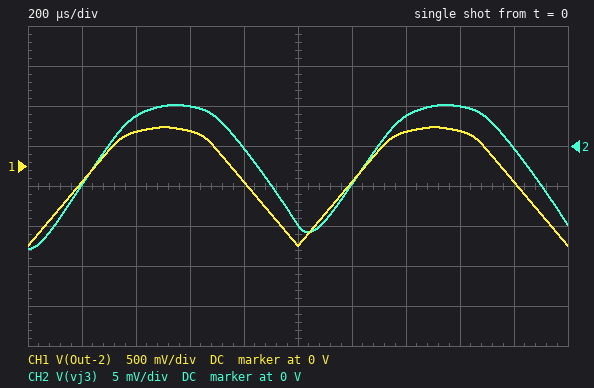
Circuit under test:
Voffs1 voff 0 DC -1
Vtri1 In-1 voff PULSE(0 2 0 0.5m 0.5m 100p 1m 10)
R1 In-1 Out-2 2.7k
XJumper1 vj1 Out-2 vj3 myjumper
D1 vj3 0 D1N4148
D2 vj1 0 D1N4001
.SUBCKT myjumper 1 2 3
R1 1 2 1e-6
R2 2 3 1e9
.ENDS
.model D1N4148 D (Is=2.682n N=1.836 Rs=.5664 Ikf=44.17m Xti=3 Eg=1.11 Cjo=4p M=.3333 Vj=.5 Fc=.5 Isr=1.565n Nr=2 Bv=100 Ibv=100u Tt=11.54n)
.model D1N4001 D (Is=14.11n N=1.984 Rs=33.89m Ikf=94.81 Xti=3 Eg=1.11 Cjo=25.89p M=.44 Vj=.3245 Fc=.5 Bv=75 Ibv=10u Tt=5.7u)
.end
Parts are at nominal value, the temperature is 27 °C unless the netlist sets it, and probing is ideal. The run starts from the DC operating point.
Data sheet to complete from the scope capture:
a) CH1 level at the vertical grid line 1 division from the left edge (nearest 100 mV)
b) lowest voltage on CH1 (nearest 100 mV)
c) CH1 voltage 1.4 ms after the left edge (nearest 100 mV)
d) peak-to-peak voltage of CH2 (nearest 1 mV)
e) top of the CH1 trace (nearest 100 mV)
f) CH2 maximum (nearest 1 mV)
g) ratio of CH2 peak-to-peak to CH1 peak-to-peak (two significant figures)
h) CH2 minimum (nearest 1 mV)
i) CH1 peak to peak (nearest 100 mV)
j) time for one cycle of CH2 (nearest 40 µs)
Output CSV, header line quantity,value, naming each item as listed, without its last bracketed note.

quantity,value
CH1 level at the vertical grid line 1 division from the left edge,-200 mV
lowest voltage on CH1,-1.0 V
CH1 voltage 1.4 ms after the left edge,400 mV
peak-to-peak voltage of CH2,18 mV
top of the CH1 trace,500 mV
CH2 maximum,5 mV
ratio of CH2 peak-to-peak to CH1 peak-to-peak,0.012
CH2 minimum,-13 mV
CH1 peak to peak,1.5 V
time for one cycle of CH2,1.00 ms
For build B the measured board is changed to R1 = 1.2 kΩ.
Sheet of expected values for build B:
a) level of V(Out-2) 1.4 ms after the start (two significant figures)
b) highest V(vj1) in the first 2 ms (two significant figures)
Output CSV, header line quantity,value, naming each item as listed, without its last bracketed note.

quantity,value
level of V(Out-2) 1.4 ms after the start,460 mV
highest V(vj1) in the first 2 ms,520 mV
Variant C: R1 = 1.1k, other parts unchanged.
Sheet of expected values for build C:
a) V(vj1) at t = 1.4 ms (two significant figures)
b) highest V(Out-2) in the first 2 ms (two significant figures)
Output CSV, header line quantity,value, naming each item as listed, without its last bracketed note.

quantity,value
V(vj1) at t = 1.4 ms,460 mV
highest V(Out-2) in the first 2 ms,530 mV
